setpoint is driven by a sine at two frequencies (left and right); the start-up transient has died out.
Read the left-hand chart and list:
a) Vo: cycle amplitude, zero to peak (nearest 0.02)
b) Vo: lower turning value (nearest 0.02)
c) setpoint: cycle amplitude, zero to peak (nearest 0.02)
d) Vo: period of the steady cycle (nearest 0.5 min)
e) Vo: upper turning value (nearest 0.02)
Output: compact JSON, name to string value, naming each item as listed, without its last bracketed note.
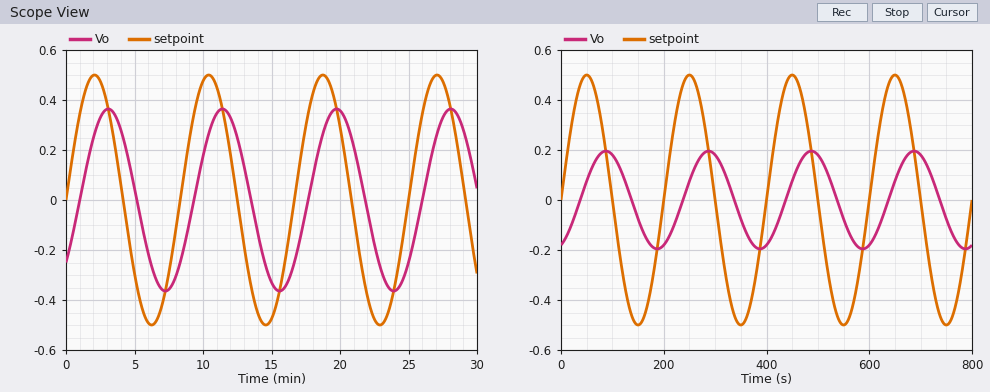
{"Vo: cycle amplitude, zero to peak": "0.36", "Vo: lower turning value": "-0.36", "setpoint: cycle amplitude, zero to peak": "0.50", "Vo: period of the steady cycle": "8.5 min", "Vo: upper turning value": "0.36"}
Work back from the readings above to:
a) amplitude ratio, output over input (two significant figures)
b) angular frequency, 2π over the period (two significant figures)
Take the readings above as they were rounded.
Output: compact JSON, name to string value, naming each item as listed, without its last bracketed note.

{"amplitude ratio, output over input": "0.72", "angular frequency, 2π over the period": "0.74 rad/min"}
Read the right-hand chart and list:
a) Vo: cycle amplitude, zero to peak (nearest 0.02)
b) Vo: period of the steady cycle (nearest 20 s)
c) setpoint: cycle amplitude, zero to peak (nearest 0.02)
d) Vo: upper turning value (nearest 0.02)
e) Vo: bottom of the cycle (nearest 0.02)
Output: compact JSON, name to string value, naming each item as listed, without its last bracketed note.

{"Vo: cycle amplitude, zero to peak": "0.20", "Vo: period of the steady cycle": "200 s", "setpoint: cycle amplitude, zero to peak": "0.50", "Vo: upper turning value": "0.20", "Vo: bottom of the cycle": "-0.20"}
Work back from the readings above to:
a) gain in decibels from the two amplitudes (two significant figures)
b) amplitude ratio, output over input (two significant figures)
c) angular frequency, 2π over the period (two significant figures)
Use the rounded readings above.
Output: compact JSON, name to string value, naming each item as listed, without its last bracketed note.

{"gain in decibels from the two amplitudes": "-8.0 dB", "amplitude ratio, output over input": "0.40", "angular frequency, 2π over the period": "0.031 rad/s"}
